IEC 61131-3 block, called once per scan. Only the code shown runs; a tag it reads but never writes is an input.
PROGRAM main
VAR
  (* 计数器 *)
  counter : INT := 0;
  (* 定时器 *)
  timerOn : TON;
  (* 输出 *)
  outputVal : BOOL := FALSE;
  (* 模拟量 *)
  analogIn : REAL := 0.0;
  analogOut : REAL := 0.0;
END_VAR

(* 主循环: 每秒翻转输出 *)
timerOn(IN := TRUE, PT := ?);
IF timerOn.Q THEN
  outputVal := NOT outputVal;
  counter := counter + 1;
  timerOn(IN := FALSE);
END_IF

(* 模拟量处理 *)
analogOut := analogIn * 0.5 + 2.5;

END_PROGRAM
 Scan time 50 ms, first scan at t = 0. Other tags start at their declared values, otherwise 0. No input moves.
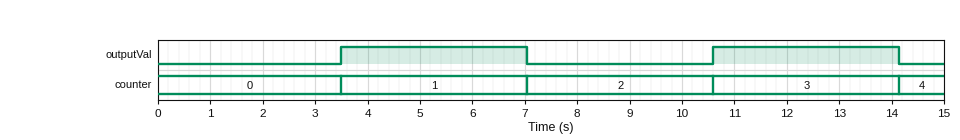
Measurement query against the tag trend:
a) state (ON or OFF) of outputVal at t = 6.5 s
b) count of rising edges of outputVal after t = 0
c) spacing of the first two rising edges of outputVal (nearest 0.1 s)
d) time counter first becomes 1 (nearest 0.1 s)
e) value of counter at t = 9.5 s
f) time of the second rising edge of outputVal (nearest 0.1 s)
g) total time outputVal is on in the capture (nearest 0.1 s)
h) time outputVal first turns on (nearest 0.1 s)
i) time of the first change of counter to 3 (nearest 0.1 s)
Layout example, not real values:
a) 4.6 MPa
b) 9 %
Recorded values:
a) ON
b) 2
c) 7.1 s
d) 3.5 s
e) 2
f) 10.6 s
g) 7.1 s
h) 3.5 s
i) 10.6 s
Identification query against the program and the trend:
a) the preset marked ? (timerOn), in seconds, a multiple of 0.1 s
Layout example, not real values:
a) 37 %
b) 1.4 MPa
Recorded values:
a) 3.5 s
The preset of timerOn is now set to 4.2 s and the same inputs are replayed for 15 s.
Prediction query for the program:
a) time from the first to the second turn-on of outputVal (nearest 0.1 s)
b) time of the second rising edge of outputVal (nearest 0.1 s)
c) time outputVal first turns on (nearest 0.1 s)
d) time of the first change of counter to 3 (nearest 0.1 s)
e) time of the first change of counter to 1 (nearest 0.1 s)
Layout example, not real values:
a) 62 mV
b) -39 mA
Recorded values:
a) 8.5 s
b) 12.7 s
c) 4.2 s
d) 12.7 s
e) 4.2 s
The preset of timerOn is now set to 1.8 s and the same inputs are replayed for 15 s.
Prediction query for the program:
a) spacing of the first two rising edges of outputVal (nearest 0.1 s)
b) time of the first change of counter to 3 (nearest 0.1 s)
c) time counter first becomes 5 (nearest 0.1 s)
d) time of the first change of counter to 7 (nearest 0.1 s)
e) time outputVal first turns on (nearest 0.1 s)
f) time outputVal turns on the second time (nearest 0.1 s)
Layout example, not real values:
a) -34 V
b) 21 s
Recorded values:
a) 3.7 s
b) 5.5 s
c) 9.2 s
d) 12.9 s
e) 1.8 s
f) 5.5 s
